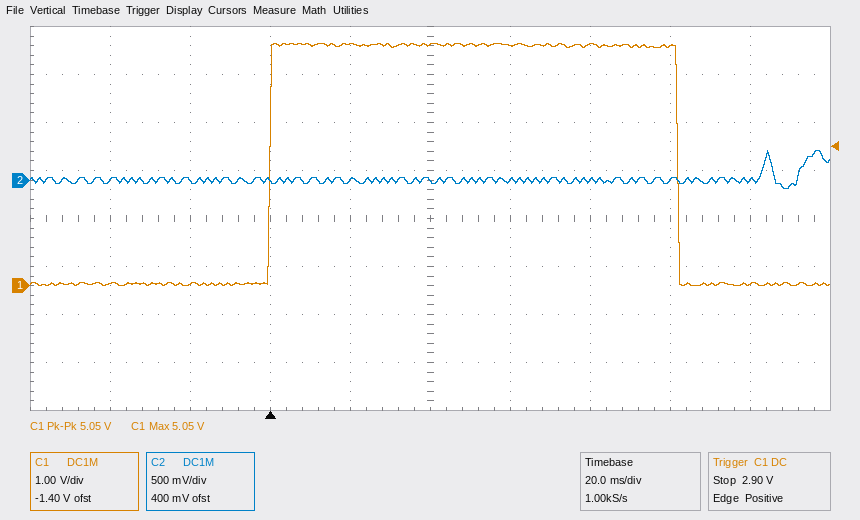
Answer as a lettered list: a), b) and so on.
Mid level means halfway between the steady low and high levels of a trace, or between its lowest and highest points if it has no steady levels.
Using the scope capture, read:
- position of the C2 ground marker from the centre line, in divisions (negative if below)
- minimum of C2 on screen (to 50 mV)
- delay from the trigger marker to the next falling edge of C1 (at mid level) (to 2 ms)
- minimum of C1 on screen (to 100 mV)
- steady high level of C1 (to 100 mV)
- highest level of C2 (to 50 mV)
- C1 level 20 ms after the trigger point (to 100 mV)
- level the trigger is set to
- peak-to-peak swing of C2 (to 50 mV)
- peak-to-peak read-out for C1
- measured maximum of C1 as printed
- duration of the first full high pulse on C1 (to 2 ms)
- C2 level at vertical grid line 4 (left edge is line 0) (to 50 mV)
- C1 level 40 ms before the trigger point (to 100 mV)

a) +0.8 div
b) -100 mV
c) 102 ms
d) 0.0 V
e) 5.0 V
f) 300 mV
g) 5.0 V
h) 2.90 V
i) 400 mV
j) 5.05 V
k) 5.05 V
l) 102 ms
m) 0 mV
n) 0.0 V
